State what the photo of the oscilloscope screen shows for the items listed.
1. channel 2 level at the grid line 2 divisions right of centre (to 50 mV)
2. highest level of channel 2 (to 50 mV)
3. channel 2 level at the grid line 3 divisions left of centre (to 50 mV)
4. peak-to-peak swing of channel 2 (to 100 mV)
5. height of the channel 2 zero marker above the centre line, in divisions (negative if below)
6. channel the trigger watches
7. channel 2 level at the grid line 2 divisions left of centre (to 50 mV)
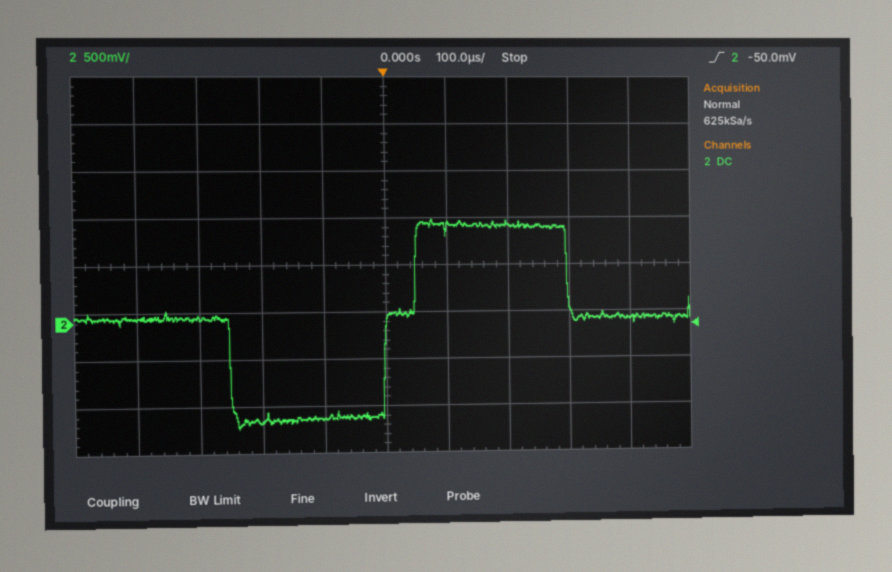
1.05 V
1.10 V
50 mV
2.20 V
-1.2 div
channel 2
-1.05 V
